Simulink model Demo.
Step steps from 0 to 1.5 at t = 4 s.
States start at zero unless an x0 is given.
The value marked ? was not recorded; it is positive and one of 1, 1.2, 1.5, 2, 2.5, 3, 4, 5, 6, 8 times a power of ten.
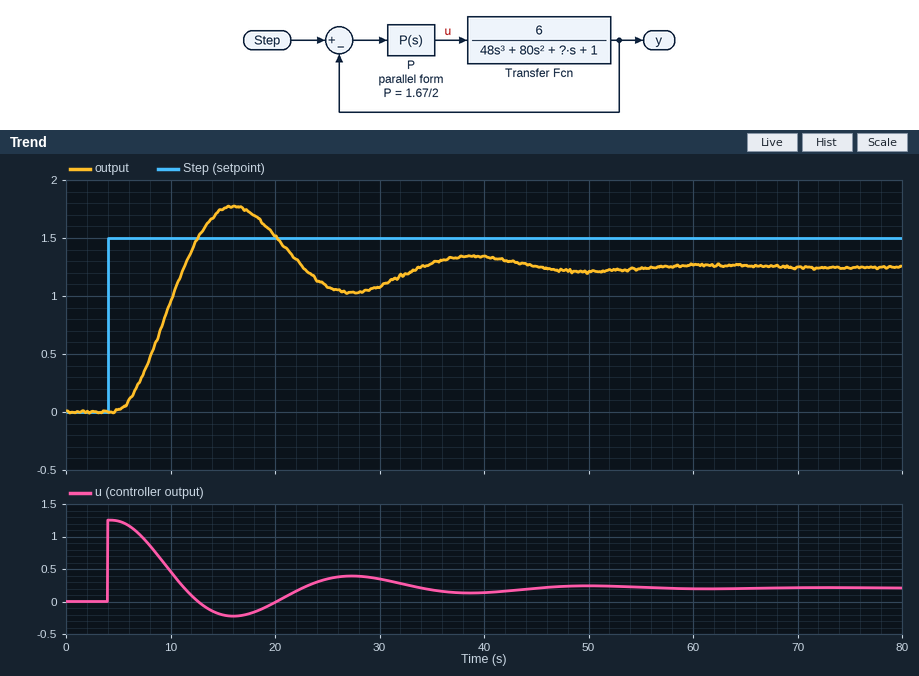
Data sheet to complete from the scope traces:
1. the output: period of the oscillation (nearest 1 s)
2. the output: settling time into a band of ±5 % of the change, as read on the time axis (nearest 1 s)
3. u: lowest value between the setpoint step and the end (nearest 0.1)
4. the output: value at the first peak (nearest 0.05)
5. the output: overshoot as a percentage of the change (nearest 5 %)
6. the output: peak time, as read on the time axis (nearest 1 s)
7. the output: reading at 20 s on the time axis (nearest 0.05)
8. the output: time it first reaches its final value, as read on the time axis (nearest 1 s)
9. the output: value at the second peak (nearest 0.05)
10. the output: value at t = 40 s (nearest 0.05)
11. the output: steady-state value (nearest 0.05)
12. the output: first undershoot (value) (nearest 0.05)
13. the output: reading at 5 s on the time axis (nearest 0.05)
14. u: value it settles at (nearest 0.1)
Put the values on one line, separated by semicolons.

23 s; 42 s; -0.2; 1.75; 40 %; 16 s; 1.50; 11 s; 1.35; 1.35; 1.25; 1.05; 0.00; 0.2
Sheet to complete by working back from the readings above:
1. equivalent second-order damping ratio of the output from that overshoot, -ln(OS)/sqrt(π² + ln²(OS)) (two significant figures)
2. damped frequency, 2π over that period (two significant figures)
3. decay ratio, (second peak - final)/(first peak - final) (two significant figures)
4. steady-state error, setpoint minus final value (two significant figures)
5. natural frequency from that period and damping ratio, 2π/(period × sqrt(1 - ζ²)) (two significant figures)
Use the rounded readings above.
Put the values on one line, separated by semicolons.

0.28; 0.27 rad/s; 0.20; 0.25; 0.28 rad/s
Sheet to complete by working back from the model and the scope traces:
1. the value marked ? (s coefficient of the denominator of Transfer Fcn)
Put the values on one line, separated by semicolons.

15
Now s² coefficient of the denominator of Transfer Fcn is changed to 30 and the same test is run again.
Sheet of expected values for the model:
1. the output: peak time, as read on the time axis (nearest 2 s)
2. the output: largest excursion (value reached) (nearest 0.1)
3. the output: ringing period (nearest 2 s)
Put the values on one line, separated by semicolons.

12 s; 1.8; 12 s
